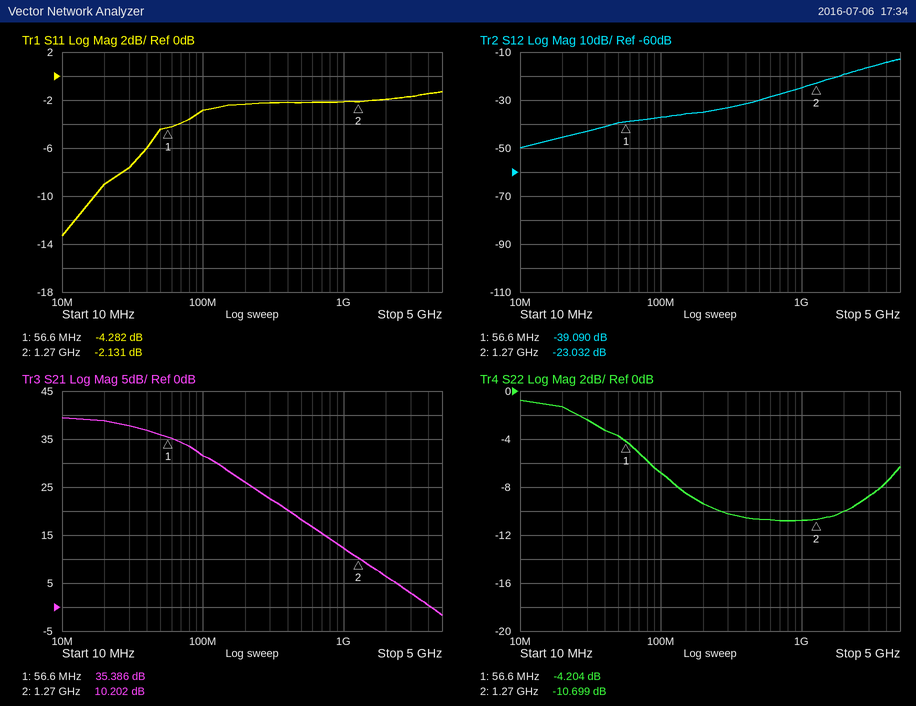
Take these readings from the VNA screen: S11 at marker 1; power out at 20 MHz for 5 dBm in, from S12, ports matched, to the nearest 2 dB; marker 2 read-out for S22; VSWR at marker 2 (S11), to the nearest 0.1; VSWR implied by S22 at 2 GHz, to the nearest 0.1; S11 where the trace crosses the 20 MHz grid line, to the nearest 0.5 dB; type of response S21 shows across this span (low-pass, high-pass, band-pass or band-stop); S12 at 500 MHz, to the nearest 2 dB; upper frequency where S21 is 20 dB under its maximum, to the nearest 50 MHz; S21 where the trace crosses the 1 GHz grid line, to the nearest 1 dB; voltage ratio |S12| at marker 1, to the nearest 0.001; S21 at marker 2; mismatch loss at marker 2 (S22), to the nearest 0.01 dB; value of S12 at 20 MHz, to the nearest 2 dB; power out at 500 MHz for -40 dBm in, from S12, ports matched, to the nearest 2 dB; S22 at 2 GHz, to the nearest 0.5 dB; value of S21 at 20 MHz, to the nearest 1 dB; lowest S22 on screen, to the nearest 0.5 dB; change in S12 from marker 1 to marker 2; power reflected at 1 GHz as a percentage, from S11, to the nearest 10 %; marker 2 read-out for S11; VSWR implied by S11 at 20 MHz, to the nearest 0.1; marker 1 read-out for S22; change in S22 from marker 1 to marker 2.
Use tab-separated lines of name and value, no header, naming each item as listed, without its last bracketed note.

S11 at marker 1	-4.282 dB
power out at 20 MHz for 5 dBm in, from S12, ports matched, to the nearest 2 dB	-40 dBm
marker 2 read-out for S22	-10.699 dB
VSWR at marker 2 (S11), to the nearest 0.1	8.2
VSWR implied by S22 at 2 GHz, to the nearest 0.1	1.9
S11 where the trace crosses the 20 MHz grid line, to the nearest 0.5 dB	-9.0 dB
type of response S21 shows across this span	low-pass
S12 at 500 MHz, to the nearest 2 dB	-30 dB
upper frequency where S21 is 20 dB under its maximum, to the nearest 50 MHz	450 MHz
S21 where the trace crosses the 1 GHz grid line, to the nearest 1 dB	12 dB
voltage ratio |S12| at marker 1, to the nearest 0.001	0.011
S21 at marker 2	10.202 dB
mismatch loss at marker 2 (S22), to the nearest 0.01 dB	0.39 dB
value of S12 at 20 MHz, to the nearest 2 dB	-46 dB
power out at 500 MHz for -40 dBm in, from S12, ports matched, to the nearest 2 dB	-70 dBm
S22 at 2 GHz, to the nearest 0.5 dB	-10.0 dB
value of S21 at 20 MHz, to the nearest 1 dB	39 dB
lowest S22 on screen, to the nearest 0.5 dB	-11.0 dB
change in S12 from marker 1 to marker 2	16.058 dB
power reflected at 1 GHz as a percentage, from S11, to the nearest 10 %	60 %
marker 2 read-out for S11	-2.131 dB
VSWR implied by S11 at 20 MHz, to the nearest 0.1	2.1
marker 1 read-out for S22	-4.204 dB
change in S22 from marker 1 to marker 2	-6.495 dB
